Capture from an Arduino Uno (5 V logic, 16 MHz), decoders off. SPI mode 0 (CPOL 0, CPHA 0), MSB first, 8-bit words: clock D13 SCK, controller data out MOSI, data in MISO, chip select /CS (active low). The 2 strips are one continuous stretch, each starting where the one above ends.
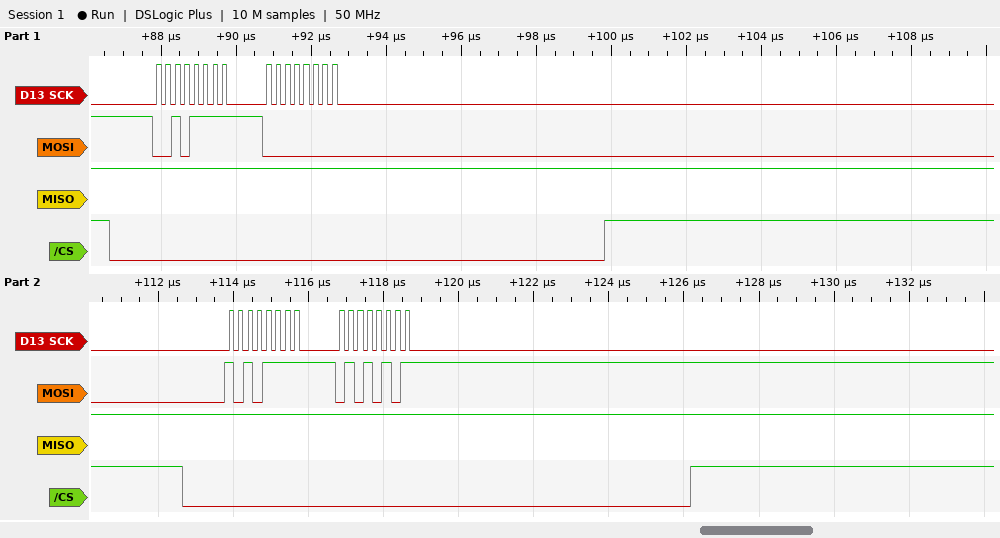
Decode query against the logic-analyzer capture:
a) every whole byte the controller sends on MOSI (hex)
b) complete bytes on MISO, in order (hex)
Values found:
2F 00 AF 55
FF FF FF FF
